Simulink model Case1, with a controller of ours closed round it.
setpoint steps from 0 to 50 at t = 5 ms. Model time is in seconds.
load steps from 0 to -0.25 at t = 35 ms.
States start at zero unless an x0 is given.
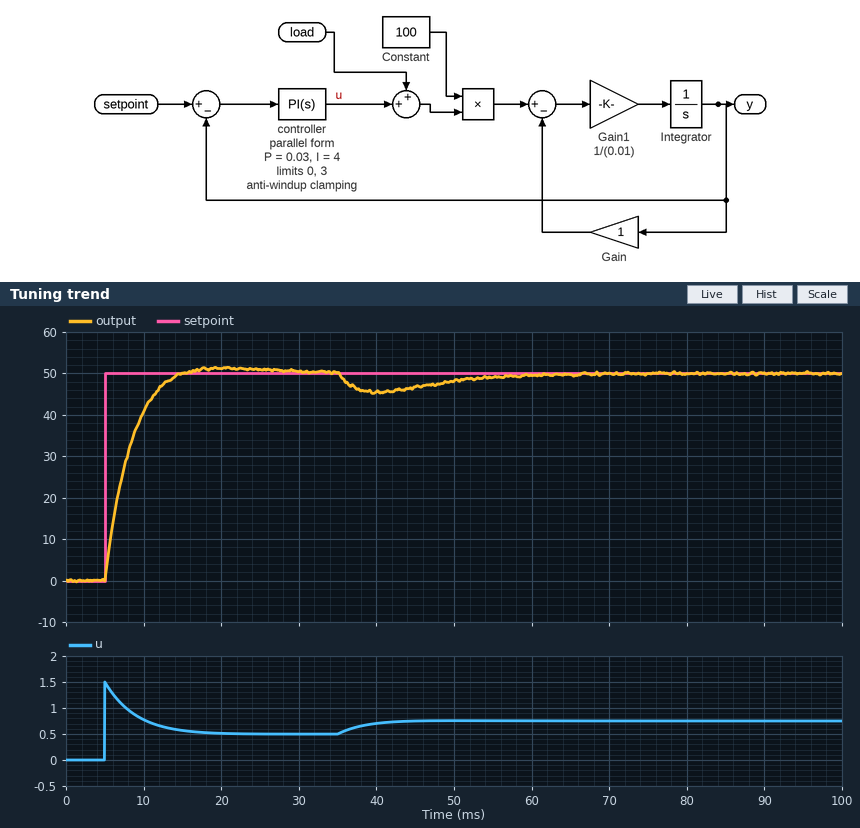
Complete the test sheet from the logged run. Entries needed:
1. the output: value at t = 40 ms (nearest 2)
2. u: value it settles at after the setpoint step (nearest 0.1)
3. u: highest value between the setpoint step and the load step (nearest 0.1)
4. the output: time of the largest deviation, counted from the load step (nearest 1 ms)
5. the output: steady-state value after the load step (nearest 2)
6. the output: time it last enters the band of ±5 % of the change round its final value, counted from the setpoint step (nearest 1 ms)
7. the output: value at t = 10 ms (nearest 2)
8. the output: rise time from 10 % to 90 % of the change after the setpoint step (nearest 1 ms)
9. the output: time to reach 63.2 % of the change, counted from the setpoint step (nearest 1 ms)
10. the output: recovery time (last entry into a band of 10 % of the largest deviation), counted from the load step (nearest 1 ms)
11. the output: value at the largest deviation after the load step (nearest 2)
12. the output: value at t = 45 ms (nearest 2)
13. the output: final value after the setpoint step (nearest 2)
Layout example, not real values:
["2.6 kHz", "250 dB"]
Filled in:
["46", "0.5", "1.5", "5 ms", "50", "8 ms", "40", "6 ms", "3 ms", "24 ms", "46", "46", "50"]
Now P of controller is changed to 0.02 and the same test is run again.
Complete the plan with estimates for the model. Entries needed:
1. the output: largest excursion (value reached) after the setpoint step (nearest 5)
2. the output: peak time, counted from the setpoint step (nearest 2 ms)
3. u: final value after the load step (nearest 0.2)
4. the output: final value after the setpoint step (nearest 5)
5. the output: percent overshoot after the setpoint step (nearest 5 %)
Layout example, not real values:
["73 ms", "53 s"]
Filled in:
["55", "14 ms", "0.8", "50", "10 %"]
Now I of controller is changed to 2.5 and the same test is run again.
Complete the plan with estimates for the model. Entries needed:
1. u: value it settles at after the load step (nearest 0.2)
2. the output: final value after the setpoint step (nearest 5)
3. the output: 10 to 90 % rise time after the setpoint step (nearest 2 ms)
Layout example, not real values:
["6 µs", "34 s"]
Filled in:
["0.8", "50", "8 ms"]
